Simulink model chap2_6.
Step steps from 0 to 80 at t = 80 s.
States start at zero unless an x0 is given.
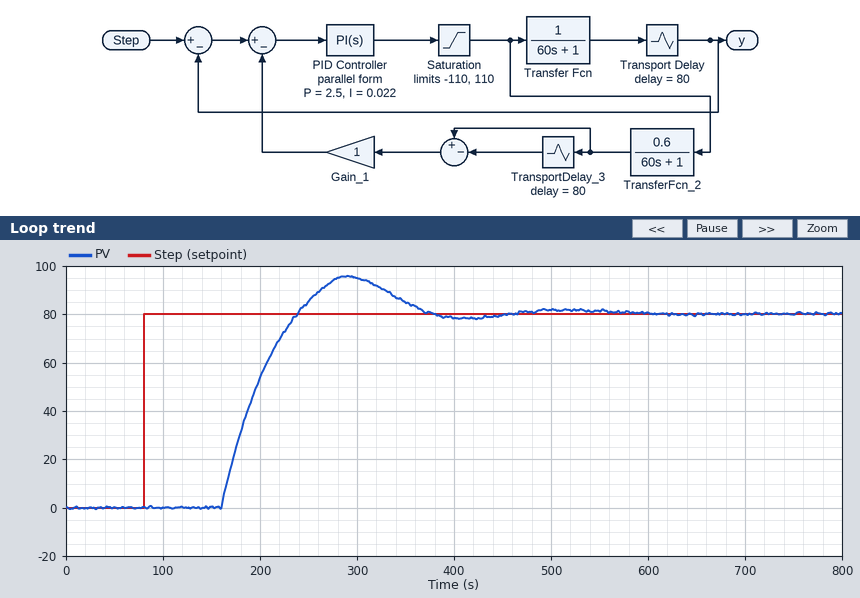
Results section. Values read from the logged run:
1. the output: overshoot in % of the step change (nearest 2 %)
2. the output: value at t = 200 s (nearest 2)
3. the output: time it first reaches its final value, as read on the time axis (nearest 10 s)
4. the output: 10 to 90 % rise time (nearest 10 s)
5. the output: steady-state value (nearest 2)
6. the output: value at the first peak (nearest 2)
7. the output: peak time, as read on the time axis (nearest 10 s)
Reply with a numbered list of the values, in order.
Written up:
1. 20 %
2. 54
3. 240 s
4. 60 s
5. 80
6. 96
7. 290 s
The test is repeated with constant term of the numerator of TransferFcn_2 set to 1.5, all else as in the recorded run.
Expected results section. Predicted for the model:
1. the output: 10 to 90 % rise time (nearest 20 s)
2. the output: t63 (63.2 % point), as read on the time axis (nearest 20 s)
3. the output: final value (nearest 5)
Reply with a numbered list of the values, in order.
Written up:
1. 220 s
2. 240 s
3. 80
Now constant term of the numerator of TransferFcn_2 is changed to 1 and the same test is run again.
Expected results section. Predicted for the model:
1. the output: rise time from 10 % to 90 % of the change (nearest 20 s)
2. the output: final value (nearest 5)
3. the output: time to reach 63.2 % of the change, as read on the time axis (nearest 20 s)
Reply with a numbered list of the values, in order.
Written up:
1. 80 s
2. 80
3. 200 s
